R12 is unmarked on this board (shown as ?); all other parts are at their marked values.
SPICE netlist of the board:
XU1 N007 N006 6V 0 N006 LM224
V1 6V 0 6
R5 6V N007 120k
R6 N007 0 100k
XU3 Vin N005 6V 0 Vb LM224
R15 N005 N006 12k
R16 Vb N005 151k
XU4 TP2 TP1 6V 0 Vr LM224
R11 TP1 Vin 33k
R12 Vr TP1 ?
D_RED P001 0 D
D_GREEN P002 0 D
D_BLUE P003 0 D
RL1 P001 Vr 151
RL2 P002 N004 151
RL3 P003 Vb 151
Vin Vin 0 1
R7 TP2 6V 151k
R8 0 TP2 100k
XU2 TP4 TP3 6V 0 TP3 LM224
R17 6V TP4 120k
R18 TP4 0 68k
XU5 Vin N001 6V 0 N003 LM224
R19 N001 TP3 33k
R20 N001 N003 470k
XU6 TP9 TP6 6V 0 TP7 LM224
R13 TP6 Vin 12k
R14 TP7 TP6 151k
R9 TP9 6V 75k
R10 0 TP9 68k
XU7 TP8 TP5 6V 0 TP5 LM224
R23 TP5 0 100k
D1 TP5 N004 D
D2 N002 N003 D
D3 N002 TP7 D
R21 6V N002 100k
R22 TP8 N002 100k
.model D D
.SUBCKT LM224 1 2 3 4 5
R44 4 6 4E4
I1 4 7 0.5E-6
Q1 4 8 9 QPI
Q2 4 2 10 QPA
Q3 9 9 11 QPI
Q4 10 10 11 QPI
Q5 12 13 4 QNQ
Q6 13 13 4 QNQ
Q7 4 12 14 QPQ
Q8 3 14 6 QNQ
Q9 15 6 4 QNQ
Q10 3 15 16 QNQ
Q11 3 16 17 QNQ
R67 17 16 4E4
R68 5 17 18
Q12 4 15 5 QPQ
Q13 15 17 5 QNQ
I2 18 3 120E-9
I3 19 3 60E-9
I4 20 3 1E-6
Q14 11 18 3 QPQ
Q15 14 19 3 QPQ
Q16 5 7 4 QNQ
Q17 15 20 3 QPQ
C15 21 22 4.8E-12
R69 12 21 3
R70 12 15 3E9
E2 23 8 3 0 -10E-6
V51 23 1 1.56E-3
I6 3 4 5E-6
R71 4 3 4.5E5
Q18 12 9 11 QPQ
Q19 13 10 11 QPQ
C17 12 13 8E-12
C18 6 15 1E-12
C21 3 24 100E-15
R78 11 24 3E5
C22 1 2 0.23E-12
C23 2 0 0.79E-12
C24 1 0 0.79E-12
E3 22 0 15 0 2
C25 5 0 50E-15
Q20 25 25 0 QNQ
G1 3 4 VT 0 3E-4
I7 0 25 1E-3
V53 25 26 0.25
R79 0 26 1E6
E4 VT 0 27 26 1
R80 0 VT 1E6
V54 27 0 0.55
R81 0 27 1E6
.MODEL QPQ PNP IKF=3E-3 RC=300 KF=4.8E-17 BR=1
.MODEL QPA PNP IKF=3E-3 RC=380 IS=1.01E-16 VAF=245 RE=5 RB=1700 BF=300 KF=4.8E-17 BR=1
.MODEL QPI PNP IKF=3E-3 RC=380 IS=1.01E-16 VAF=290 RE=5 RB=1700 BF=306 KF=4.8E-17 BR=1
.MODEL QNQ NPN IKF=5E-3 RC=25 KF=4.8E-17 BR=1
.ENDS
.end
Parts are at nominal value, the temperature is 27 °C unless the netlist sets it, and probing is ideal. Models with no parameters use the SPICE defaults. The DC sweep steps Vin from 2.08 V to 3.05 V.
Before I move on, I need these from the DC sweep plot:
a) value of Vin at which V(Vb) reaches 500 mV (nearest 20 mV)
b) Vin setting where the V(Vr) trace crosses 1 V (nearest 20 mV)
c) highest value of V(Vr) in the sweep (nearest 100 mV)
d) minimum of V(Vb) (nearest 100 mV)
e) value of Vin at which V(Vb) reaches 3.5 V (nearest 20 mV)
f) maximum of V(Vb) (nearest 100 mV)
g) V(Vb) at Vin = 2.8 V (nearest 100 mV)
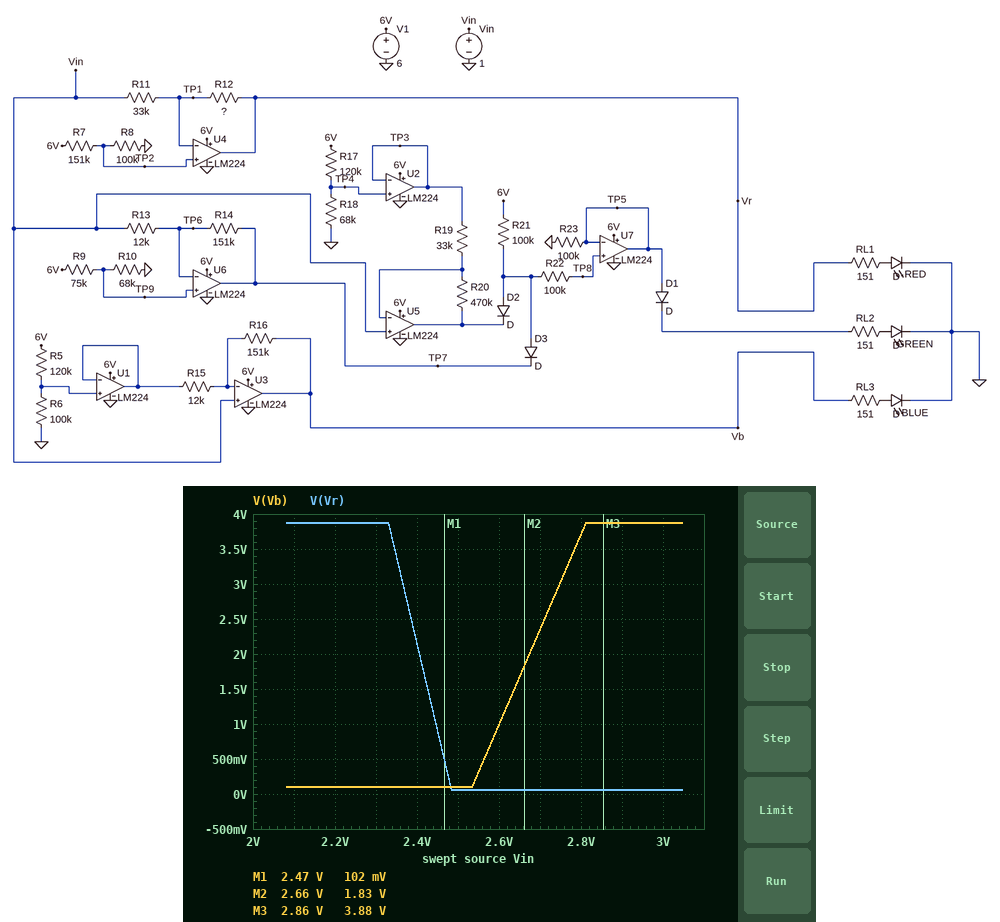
2.56 V
2.44 V
3.9 V
100 mV
2.78 V
3.9 V
3.7 V
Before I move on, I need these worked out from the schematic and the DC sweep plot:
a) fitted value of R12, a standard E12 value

820 kΩ
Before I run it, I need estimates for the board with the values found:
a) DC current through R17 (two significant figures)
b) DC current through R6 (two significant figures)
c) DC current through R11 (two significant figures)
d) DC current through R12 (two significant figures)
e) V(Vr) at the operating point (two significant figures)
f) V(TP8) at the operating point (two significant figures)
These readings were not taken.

32 µA
27 µA
3.4 µA
3.4 µA
3.9 V
1.2 V
